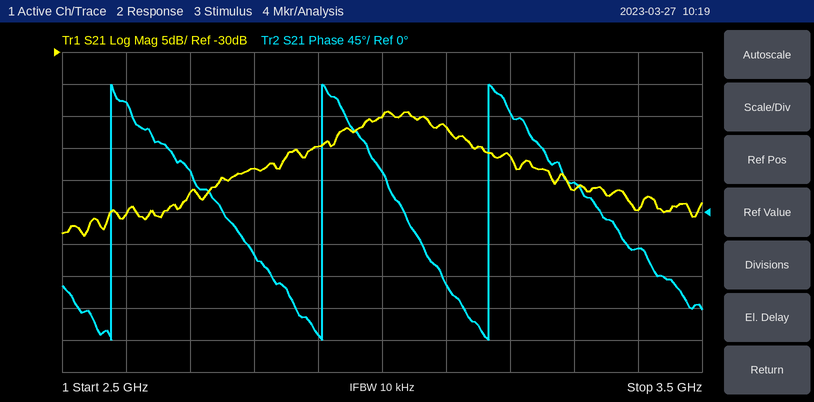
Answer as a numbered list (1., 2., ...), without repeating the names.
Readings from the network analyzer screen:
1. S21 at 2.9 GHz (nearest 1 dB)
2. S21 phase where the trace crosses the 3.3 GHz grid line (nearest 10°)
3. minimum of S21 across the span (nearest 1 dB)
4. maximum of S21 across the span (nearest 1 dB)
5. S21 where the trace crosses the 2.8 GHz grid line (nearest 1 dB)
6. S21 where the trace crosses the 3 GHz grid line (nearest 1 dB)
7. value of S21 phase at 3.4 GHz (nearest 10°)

1. -45 dB
2. 40°
3. -59 dB
4. -39 dB
5. -48 dB
6. -40 dB
7. -50°
